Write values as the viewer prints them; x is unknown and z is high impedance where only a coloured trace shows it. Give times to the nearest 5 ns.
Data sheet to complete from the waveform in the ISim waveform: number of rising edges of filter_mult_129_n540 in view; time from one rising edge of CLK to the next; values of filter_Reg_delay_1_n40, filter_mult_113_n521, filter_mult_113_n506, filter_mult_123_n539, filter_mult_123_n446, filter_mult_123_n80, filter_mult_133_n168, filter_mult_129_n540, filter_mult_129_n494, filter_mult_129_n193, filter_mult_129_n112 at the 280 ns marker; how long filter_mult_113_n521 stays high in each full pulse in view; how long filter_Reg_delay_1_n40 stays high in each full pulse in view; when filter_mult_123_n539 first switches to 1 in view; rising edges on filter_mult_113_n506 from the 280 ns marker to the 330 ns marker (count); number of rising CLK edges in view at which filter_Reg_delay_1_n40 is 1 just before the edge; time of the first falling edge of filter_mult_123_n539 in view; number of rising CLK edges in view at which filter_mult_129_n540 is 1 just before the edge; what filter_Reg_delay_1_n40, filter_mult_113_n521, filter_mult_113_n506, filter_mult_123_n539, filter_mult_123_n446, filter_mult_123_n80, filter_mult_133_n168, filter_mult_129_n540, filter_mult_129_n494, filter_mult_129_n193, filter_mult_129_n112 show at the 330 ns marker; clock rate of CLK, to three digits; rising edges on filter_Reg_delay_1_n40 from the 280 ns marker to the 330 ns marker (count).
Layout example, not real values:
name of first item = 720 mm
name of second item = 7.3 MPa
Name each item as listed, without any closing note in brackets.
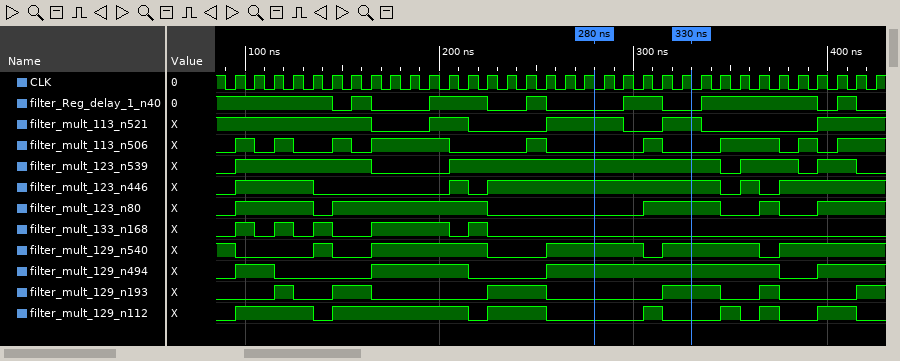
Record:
number of rising edges of filter_mult_129_n540 in view = 5
time from one rising edge of CLK to the next = 10 ns
values of filter_Reg_delay_1_n40, filter_mult_113_n521, filter_mult_113_n506, filter_mult_123_n539, filter_mult_123_n446, filter_mult_123_n80, filter_mult_133_n168, filter_mult_129_n540, filter_mult_129_n494, filter_mult_129_n193, filter_mult_129_n112 at the 280 ns marker = filter_Reg_delay_1_n40=0, filter_mult_113_n521=1, filter_mult_113_n506=0, filter_mult_123_n539=1, filter_mult_123_n446=1, filter_mult_123_n80=0, filter_mult_133_n168=0, filter_mult_129_n540=1, filter_mult_129_n494=1, filter_mult_129_n193=0, filter_mult_129_n112=0
how long filter_mult_113_n521 stays high in each full pulse in view = 20 ns, 40 ns, 20 ns
how long filter_Reg_delay_1_n40 stays high in each full pulse in view = 10 ns, 30 ns, 10 ns, 20 ns, 60 ns, 10 ns
when filter_mult_123_n539 first switches to 1 in view = 95 ns
rising edges on filter_mult_113_n506 from the 280 ns marker to the 330 ns marker = 1
number of rising CLK edges in view at which filter_Reg_delay_1_n40 is 1 just before the edge = 20
time of the first falling edge of filter_mult_123_n539 in view = 165 ns
number of rising CLK edges in view at which filter_mult_129_n540 is 1 just before the edge = 23
what filter_Reg_delay_1_n40, filter_mult_113_n521, filter_mult_113_n506, filter_mult_123_n539, filter_mult_123_n446, filter_mult_123_n80, filter_mult_133_n168, filter_mult_129_n540, filter_mult_129_n494, filter_mult_129_n193, filter_mult_129_n112 show at the 330 ns marker = filter_Reg_delay_1_n40=0, filter_mult_113_n521=1, filter_mult_113_n506=0, filter_mult_123_n539=1, filter_mult_123_n446=1, filter_mult_123_n80=1, filter_mult_133_n168=0, filter_mult_129_n540=1, filter_mult_129_n494=1, filter_mult_129_n193=1, filter_mult_129_n112=0
clock rate of CLK, to three digits = 100 MHz
rising edges on filter_Reg_delay_1_n40 from the 280 ns marker to the 330 ns marker = 1
